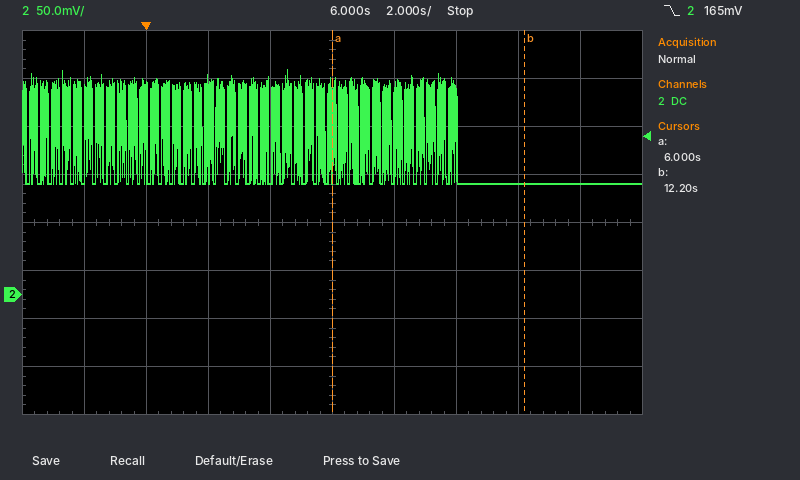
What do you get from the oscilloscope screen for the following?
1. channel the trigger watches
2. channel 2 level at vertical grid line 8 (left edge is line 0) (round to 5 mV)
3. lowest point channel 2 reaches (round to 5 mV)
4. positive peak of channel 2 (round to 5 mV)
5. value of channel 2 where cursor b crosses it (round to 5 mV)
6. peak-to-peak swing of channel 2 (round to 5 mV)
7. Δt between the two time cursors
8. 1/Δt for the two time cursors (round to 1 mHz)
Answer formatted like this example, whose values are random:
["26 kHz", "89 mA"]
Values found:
["channel 2", "115 mV", "115 mV", "235 mV", "115 mV", "120 mV", "6.2 s", "161 mHz"]
